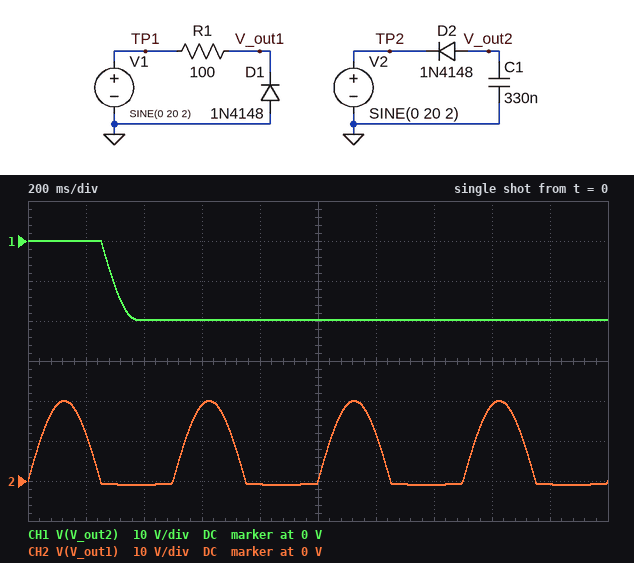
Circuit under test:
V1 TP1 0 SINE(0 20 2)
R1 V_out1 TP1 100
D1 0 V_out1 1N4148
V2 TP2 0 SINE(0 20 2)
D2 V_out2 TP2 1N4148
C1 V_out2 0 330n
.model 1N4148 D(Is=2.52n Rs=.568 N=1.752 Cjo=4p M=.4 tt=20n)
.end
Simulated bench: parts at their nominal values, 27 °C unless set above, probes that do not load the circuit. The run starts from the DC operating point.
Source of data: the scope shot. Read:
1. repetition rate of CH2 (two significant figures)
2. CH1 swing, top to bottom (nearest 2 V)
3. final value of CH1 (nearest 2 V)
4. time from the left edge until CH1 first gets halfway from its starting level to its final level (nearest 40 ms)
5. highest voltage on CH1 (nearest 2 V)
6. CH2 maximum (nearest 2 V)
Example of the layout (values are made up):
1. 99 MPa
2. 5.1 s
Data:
1. 2.0 Hz
2. 20 V
3. -20 V
4. 280 ms
5. 0 V
6. 20 V
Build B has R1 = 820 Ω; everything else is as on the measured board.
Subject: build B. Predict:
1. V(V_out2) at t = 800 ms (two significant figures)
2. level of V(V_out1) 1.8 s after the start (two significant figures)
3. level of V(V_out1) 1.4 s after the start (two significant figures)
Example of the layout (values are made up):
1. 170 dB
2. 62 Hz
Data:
1. -20 V
2. -710 mV
3. -740 mV
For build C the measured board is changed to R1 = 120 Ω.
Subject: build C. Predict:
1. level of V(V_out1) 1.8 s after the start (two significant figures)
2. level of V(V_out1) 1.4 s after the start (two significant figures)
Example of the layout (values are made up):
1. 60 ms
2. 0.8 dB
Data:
1. -840 mV
2. -900 mV
